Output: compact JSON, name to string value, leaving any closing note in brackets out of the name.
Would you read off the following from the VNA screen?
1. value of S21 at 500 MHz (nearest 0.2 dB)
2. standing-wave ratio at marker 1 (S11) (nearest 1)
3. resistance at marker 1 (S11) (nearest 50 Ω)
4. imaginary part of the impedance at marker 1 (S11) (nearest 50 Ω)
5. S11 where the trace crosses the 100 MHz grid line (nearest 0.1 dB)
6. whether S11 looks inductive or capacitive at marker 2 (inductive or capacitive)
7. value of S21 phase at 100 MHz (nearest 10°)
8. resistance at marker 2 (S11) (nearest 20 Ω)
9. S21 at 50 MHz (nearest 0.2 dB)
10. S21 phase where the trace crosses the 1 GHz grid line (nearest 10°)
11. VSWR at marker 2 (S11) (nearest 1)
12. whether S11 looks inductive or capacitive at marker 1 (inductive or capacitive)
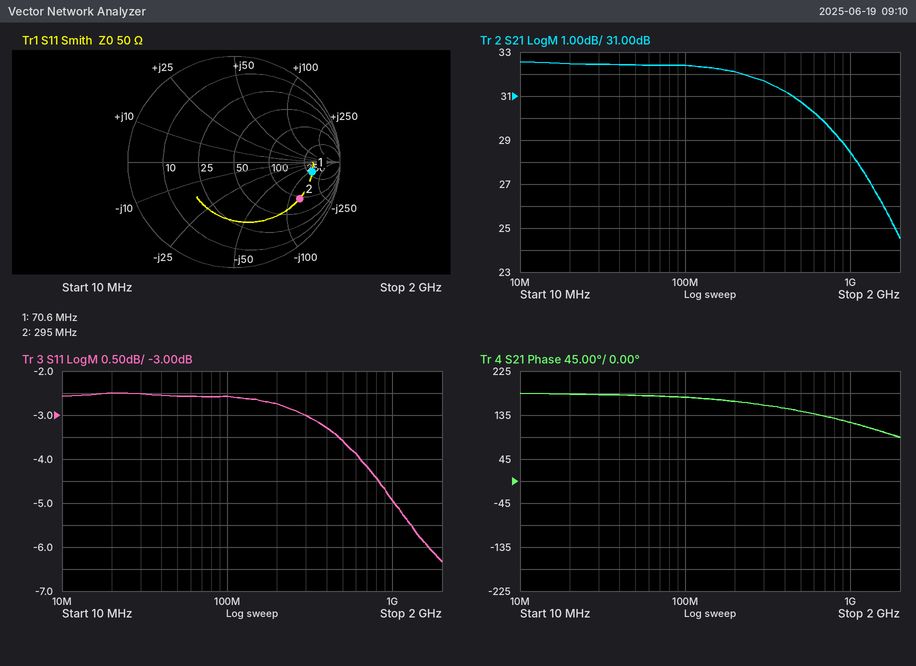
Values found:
{"value of S21 at 500 MHz": "30.8 dB", "standing-wave ratio at marker 1 (S11)": "7", "resistance at marker 1 (S11)": "300 Ω", "imaginary part of the impedance at marker 1 (S11)": "-100 Ω", "S11 where the trace crosses the 100 MHz grid line": "-2.6 dB", "whether S11 looks inductive or capacitive at marker 2": "capacitive", "value of S21 phase at 100 MHz": "170°", "resistance at marker 2 (S11)": "100 Ω", "S21 at 50 MHz": "32.4 dB", "S21 phase where the trace crosses the 1 GHz grid line": "120°", "VSWR at marker 2 (S11)": "6", "whether S11 looks inductive or capacitive at marker 1": "capacitive"}
